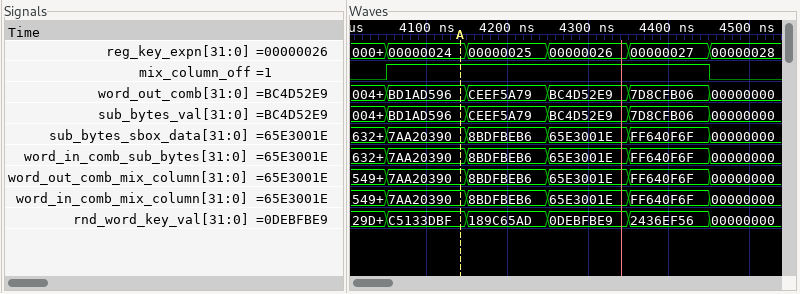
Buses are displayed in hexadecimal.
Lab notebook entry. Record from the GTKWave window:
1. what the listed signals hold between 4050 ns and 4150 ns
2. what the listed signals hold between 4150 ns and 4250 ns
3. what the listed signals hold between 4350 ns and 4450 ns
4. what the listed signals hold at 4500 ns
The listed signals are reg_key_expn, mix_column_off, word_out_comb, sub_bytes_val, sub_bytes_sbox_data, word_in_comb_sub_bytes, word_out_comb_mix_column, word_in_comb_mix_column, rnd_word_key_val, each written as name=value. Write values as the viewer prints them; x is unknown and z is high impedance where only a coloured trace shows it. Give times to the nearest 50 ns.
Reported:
reg_key_expn=00000024, mix_column_off=1, word_out_comb=BD1AD596, sub_bytes_val=BD1AD596, sub_bytes_sbox_data=7AA20390, word_in_comb_sub_bytes=7AA20390, word_out_comb_mix_column=7AA20390, word_in_comb_mix_column=7AA20390, rnd_word_key_val=C5133DBF
reg_key_expn=00000025, mix_column_off=1, word_out_comb=CEEF5A79, sub_bytes_val=CEEF5A79, sub_bytes_sbox_data=8BDFBEB6, word_in_comb_sub_bytes=8BDFBEB6, word_out_comb_mix_column=8BDFBEB6, word_in_comb_mix_column=8BDFBEB6, rnd_word_key_val=189C65AD
reg_key_expn=00000027, mix_column_off=1, word_out_comb=7D8CFB06, sub_bytes_val=7D8CFB06, sub_bytes_sbox_data=FF640F6F, word_in_comb_sub_bytes=FF640F6F, word_out_comb_mix_column=FF640F6F, word_in_comb_mix_column=FF640F6F, rnd_word_key_val=2436EF56
reg_key_expn=00000028, mix_column_off=0, word_out_comb=00000000, sub_bytes_val=00000000, sub_bytes_sbox_data=00000000, word_in_comb_sub_bytes=00000000, word_out_comb_mix_column=00000000, word_in_comb_mix_column=00000000, rnd_word_key_val=00000000
